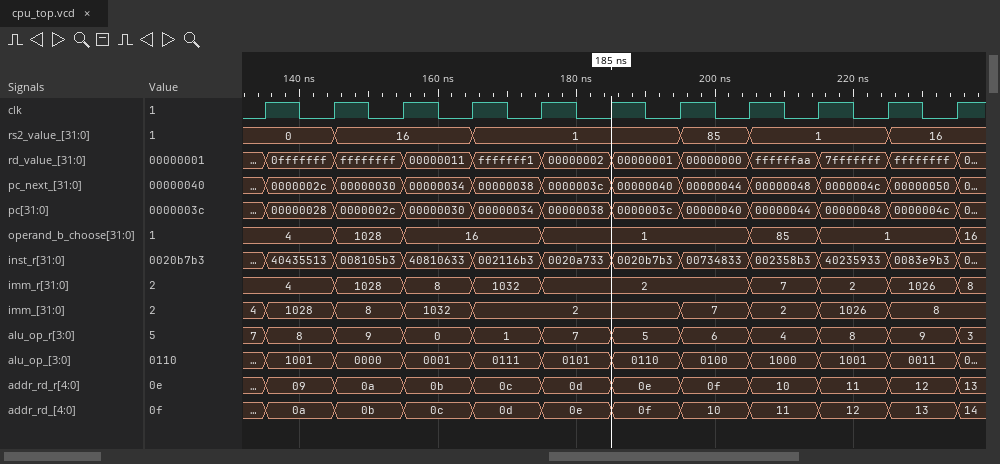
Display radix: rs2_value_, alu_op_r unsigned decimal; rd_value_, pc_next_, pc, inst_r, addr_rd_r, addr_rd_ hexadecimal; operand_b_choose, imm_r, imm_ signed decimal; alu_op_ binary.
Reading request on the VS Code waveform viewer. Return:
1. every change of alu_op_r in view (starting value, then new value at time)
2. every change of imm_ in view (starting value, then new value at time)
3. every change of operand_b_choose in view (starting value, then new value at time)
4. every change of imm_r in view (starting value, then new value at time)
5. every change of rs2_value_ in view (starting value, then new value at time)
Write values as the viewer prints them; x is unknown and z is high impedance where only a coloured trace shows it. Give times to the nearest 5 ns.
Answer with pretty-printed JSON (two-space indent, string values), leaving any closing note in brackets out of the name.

{
  "every change of alu_op_r in view": "7, 8 at 135 ns, 9 at 145 ns, 0 at 155 ns, 1 at 165 ns, 7 at 175 ns, 5 at 185 ns, 6 at 195 ns, 4 at 205 ns, 8 at 215 ns, 9 at 225 ns, 3 at 235 ns",
  "every change of imm_ in view": "4, 1028 at 135 ns, 8 at 145 ns, 1032 at 155 ns, 2 at 165 ns, 7 at 195 ns, 2 at 205 ns, 1026 at 215 ns, 8 at 225 ns",
  "every change of operand_b_choose in view": "4, 1028 at 145 ns, 16 at 155 ns, 1 at 175 ns, 85 at 205 ns, 1 at 215 ns, 16 at 235 ns",
  "every change of imm_r in view": "4, 1028 at 145 ns, 8 at 155 ns, 1032 at 165 ns, 2 at 175 ns, 7 at 205 ns, 2 at 215 ns, 1026 at 225 ns, 8 at 235 ns",
  "every change of rs2_value_ in view": "0, 16 at 145 ns, 1 at 165 ns, 85 at 195 ns, 1 at 205 ns, 16 at 225 ns"
}
